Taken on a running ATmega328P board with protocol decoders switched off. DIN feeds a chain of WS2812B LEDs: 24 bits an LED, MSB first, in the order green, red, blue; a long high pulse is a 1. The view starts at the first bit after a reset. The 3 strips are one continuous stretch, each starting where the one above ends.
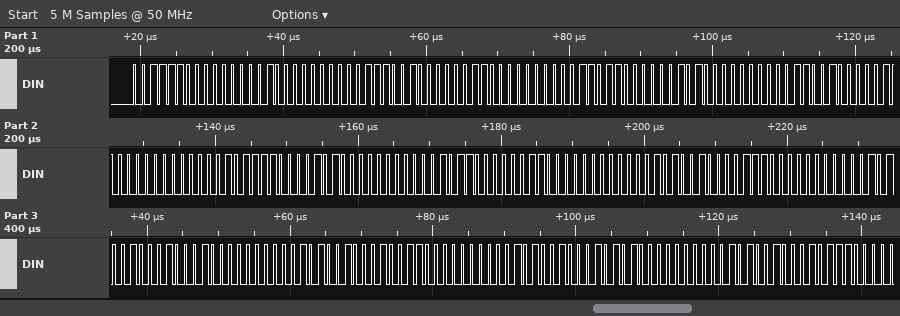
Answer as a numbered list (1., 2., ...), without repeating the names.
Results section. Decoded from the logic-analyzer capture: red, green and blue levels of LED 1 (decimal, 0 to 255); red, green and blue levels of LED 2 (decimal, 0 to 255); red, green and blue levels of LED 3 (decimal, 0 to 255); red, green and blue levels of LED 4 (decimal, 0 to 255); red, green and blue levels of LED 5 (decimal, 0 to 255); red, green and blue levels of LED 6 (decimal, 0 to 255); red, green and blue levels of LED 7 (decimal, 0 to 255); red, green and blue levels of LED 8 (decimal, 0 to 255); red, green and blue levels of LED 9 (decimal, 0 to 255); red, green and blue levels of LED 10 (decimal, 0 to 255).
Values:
1. 1, 60, 0
2. 3, 57, 0
3. 5, 54, 0
4. 8, 50, 0
5. 10, 47, 0
6. 12, 44, 0
7. 14, 41, 0
8. 17, 41, 0
9. 19, 41, 0
10. 21, 41, 0
